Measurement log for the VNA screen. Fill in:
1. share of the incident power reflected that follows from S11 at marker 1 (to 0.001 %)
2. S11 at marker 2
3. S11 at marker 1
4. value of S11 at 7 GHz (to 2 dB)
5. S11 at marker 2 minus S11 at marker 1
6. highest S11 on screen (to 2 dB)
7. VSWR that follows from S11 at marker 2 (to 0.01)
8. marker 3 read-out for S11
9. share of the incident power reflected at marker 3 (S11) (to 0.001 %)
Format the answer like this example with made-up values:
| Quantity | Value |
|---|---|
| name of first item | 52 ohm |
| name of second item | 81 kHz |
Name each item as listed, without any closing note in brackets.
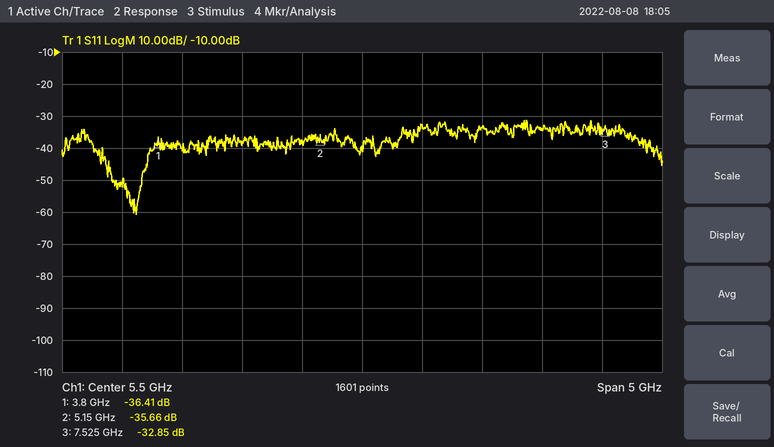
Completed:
| Quantity | Value |
|---|---|
| share of the incident power reflected that follows from S11 at marker 1 | 0.023 % |
| S11 at marker 2 | -35.66 dB |
| S11 at marker 1 | -36.41 dB |
| value of S11 at 7 GHz | -34 dB |
| S11 at marker 2 minus S11 at marker 1 | 0.75 dB |
| highest S11 on screen | -32 dB |
| VSWR that follows from S11 at marker 2 | 1.03 |
| marker 3 read-out for S11 | -32.85 dB |
| share of the incident power reflected at marker 3 (S11) | 0.052 % |
